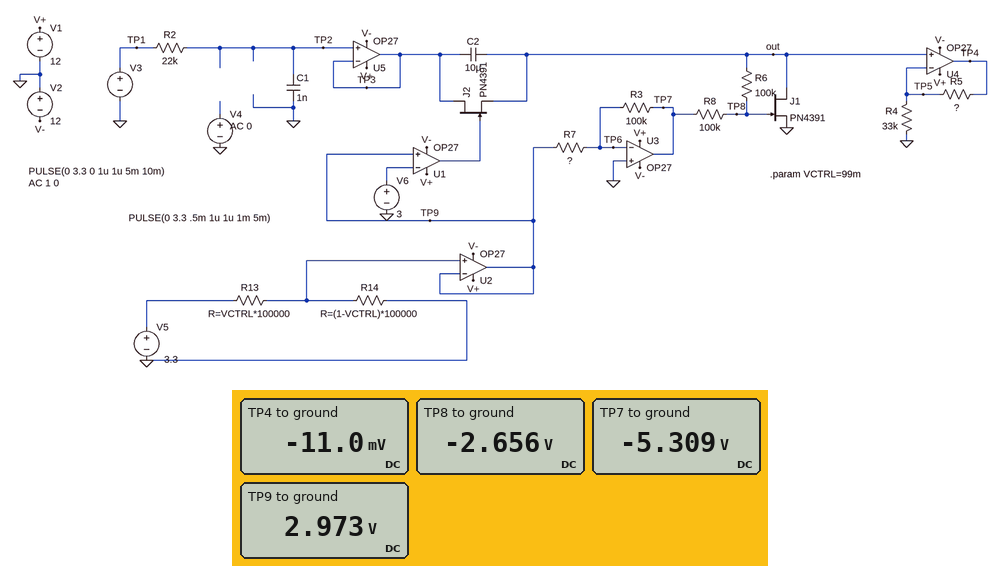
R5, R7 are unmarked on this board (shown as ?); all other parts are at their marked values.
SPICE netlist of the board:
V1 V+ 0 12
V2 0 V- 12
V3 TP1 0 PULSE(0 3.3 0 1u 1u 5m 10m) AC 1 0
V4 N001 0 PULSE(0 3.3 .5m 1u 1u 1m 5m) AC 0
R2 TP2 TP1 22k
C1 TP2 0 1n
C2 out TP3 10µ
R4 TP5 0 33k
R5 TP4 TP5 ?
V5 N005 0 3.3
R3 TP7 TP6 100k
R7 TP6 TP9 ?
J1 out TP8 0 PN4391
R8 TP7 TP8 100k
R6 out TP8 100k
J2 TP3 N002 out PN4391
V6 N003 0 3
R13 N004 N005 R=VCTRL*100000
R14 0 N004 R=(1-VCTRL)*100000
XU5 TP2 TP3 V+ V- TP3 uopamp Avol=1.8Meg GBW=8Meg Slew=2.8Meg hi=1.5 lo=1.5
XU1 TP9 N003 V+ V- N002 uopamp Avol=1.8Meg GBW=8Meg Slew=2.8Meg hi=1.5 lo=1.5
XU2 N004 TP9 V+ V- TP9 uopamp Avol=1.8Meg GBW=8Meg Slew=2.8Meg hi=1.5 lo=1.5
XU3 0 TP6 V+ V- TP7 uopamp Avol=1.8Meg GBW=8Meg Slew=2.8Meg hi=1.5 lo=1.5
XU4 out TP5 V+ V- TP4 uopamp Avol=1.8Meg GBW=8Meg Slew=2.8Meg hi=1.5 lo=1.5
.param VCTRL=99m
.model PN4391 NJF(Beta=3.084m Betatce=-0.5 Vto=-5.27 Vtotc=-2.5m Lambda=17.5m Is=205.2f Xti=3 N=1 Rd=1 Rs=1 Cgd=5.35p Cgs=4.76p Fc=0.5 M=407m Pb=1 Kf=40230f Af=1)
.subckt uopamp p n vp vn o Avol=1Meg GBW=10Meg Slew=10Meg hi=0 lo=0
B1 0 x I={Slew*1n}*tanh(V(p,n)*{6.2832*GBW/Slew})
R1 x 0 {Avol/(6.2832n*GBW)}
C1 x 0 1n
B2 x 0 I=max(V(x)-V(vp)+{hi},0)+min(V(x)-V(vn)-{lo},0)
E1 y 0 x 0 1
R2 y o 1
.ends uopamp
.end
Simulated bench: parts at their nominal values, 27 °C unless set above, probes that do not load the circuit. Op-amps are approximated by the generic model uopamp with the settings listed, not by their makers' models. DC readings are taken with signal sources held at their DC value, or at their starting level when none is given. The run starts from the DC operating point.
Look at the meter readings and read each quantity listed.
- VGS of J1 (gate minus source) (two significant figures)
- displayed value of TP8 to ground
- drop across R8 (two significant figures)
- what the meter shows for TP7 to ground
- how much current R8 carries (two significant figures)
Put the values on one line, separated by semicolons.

-2.7 V; -2.656 V; 2.7 V; -5.309 V; 27 µA
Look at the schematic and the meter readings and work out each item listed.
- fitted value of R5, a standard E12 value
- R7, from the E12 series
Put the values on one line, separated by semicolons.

180 kΩ; 56 kΩ
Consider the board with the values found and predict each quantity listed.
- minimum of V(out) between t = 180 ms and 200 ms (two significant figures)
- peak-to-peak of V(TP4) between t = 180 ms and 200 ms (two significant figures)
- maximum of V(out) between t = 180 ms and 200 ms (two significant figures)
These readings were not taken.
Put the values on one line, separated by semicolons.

-2.9 V; 21 V; 2.9 V
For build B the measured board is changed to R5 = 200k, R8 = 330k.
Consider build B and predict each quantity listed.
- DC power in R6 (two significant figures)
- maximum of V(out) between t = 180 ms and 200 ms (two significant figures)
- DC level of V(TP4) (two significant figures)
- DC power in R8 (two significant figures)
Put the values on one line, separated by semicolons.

15 µW; 2.8 V; -3.7 mV; 50 µW
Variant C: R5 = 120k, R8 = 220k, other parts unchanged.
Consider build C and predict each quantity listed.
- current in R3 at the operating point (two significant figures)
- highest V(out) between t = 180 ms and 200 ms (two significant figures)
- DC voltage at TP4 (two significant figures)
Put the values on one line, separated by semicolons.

53 µA; 2.8 V; -3.6 mV
